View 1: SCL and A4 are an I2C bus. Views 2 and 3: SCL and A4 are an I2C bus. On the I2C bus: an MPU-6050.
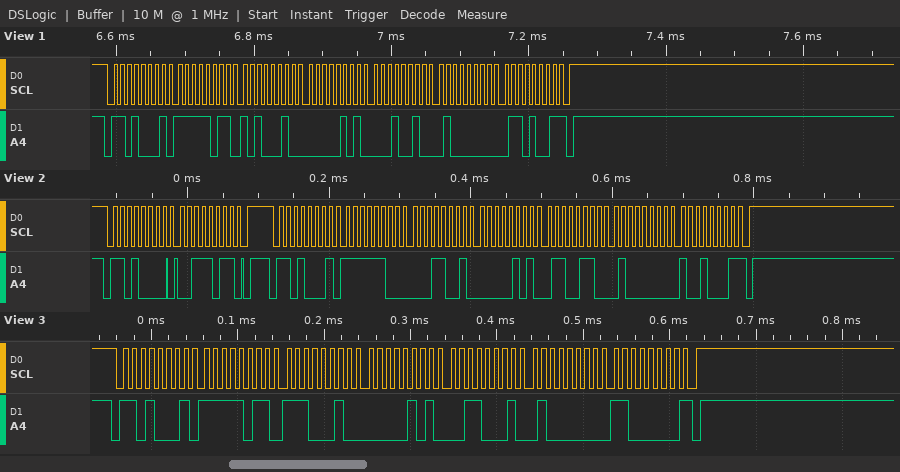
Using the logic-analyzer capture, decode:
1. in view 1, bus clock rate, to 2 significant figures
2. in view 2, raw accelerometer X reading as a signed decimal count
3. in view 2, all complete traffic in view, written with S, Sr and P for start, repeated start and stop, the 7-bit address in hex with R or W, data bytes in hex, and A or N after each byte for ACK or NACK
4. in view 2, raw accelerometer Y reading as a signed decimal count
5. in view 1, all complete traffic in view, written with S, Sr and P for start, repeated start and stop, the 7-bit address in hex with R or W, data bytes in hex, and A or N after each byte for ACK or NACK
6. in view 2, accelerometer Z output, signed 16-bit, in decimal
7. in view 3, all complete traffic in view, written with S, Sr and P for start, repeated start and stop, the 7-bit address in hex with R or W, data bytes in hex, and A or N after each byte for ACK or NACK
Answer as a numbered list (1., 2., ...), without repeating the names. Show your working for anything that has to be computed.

1. 100 kHz
2. 0xFC19 = -999
3. S 68W A 3B A P S 68R A FC A 19 A 05 A 66 A 40 A 91 N P
4. 0x0566 = 1382
5. S 68R A FB A A2 A 05 A 12 A 40 A 69 N P
6. 0x4091 = 16529
7. S 68R A FB A E2 A 05 A 31 A 40 A C0 N P
